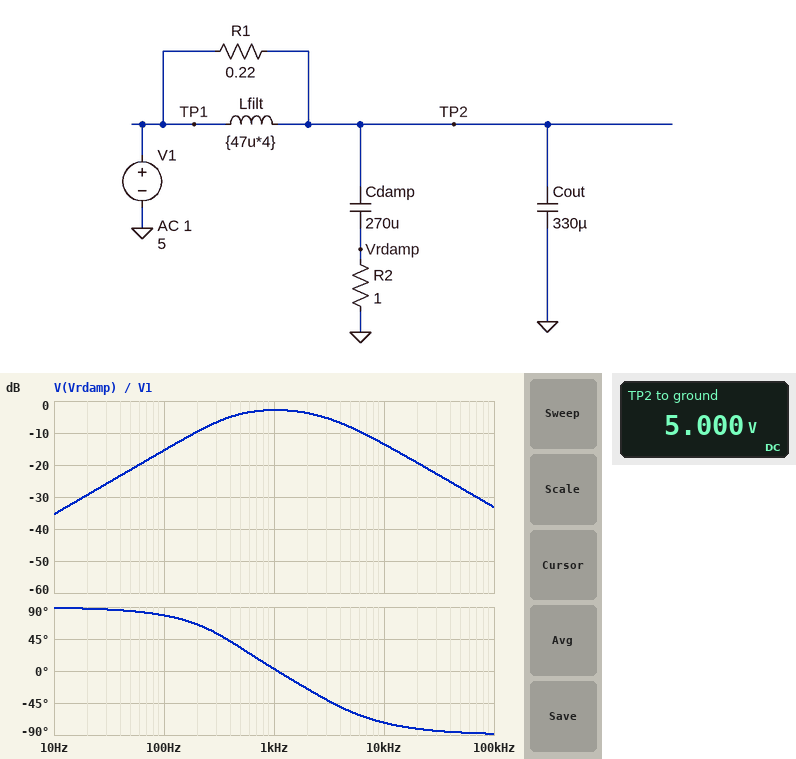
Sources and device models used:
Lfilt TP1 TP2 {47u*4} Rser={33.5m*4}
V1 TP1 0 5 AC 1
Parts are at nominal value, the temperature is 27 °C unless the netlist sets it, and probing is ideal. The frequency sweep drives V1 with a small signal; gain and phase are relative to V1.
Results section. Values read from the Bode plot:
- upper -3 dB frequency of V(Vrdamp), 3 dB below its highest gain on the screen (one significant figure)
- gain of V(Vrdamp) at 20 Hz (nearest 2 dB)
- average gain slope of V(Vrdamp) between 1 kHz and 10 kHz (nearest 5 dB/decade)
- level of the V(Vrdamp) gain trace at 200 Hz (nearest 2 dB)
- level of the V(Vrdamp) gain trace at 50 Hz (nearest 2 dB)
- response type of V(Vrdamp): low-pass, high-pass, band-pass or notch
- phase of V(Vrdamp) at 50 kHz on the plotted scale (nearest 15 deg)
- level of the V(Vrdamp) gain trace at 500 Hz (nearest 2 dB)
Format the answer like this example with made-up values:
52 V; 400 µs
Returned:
3 kHz; -30 dB; -10 dB/decade; -10 dB; -22 dB; band-pass; -90 deg; -4 dB
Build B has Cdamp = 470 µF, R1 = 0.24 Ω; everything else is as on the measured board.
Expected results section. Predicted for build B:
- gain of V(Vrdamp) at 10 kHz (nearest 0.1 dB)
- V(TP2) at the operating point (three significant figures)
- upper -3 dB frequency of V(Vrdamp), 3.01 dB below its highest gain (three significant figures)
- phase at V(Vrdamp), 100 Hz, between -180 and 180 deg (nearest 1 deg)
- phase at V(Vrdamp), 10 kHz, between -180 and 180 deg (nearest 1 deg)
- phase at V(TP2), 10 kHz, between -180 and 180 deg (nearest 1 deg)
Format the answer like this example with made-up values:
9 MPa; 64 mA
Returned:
-14.2 dB; 5.00 V; 2.74 kHz; 71 deg; -75 deg; -77 deg
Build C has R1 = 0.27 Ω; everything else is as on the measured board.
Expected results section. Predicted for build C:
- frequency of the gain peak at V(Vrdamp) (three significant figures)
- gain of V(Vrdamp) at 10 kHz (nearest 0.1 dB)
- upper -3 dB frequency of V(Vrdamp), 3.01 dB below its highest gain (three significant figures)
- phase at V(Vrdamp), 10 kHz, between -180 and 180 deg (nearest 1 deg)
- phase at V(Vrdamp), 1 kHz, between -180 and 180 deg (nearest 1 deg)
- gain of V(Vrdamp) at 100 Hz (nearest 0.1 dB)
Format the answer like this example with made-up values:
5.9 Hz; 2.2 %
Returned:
883 Hz; -15.2 dB; 2.83 kHz; -75 deg; -2 deg; -15.4 dB
